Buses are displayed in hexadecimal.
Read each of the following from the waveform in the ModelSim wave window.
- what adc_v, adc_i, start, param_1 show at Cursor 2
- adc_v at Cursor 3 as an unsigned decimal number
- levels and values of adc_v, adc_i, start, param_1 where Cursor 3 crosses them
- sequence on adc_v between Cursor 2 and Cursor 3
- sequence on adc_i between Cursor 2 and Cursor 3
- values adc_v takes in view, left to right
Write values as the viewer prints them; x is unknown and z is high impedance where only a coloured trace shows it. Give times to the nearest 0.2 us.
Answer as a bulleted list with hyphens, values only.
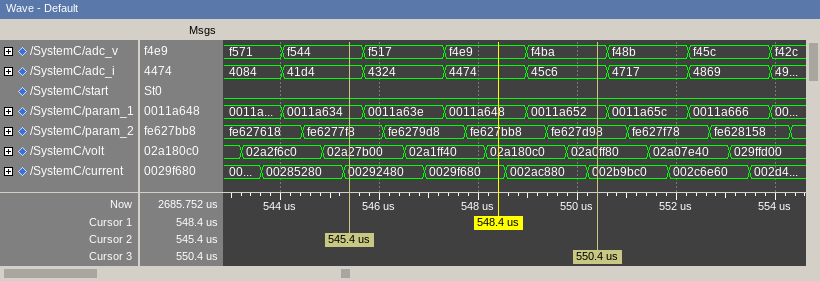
- adc_v=f544, adc_i=41d4, start=0, param_1=0011a634
- 62650
- adc_v=f4ba, adc_i=45c6, start=0, param_1=0011a652
- f544, f517, f4e9, f4ba
- 41d4, 4324, 4474, 45c6
- f571, f544, f517, f4e9, f4ba, f48b, f45c, f42c
